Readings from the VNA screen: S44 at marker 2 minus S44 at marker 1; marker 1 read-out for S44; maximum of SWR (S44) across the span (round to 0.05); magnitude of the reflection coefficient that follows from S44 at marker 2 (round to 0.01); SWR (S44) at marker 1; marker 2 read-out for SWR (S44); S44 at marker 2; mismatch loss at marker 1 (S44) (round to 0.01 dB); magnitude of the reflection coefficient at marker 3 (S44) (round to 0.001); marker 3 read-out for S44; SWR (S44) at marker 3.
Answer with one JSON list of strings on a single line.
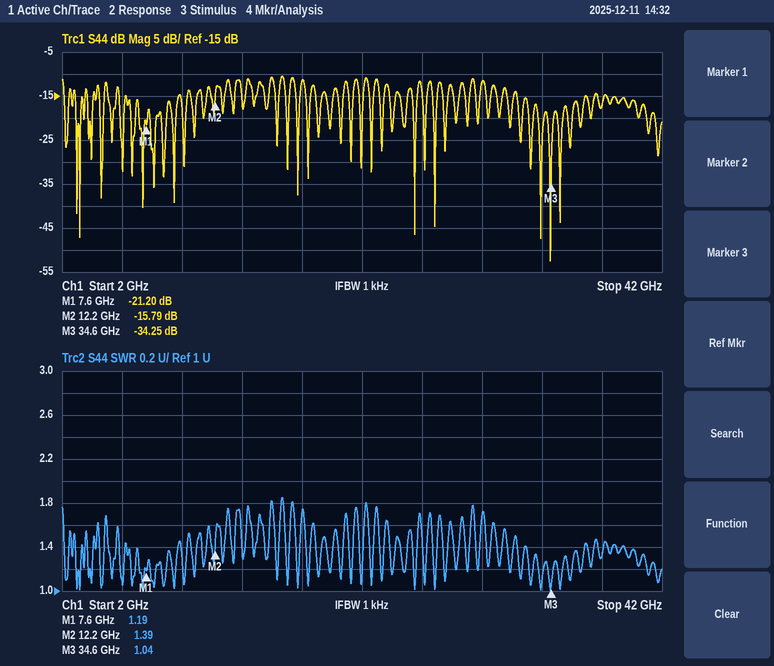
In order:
["5.41 dB", "-21.20 dB", "1.85", "0.16", "1.19", "1.39", "-15.79 dB", "0.03 dB", "0.019", "-34.25 dB", "1.04"]
